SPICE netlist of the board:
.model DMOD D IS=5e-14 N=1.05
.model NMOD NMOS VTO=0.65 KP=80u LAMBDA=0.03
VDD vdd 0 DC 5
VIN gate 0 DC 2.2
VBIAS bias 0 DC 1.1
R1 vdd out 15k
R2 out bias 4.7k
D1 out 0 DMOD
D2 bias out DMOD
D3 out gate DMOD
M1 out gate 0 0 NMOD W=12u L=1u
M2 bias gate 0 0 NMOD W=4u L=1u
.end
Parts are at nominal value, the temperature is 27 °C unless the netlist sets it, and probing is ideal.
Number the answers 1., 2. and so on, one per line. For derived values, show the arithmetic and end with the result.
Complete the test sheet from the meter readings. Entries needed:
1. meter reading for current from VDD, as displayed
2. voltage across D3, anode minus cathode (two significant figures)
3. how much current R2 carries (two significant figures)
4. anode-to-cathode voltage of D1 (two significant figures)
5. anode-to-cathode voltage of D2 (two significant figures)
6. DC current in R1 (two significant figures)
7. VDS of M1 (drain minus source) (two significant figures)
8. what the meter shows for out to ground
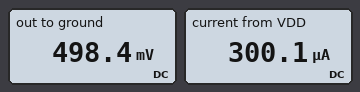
1. 300.1 µA
2. 498.4 mV - 2.2 V = -1.7 V
3. (1.1 V - 498.4 mV) / 4.7 kΩ = 130 µA
4. 498.4 mV = 500 mV
5. 1.1 V - 498.4 mV = 600 mV
6. (5 V - 498.4 mV) / 15 kΩ = 300 µA
7. 498.4 mV = 500 mV
8. 498.4 mV
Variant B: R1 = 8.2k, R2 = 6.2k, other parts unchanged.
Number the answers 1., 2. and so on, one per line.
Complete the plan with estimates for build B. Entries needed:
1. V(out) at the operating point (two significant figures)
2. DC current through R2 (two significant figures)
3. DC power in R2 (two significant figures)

1. 540 mV
2. 91 µA
3. 51 µW
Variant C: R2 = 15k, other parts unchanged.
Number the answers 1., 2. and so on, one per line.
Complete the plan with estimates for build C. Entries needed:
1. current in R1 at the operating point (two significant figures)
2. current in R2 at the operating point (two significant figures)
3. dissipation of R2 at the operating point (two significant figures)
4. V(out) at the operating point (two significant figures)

1. 300 µA
2. 41 µA
3. 25 µW
4. 490 mV
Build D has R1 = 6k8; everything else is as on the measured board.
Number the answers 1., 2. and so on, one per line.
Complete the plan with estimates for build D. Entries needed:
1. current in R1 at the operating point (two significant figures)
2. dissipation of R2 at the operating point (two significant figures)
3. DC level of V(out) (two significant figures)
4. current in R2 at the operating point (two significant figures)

1. 650 µA
2. 59 µW
3. 570 mV
4. 110 µA
